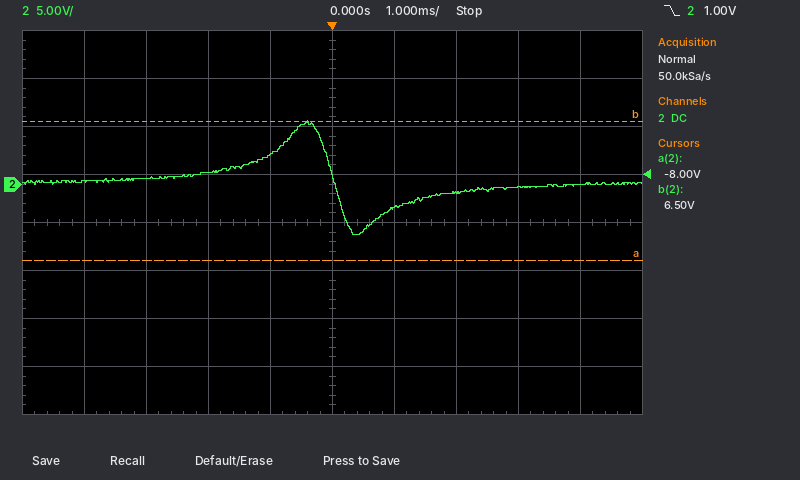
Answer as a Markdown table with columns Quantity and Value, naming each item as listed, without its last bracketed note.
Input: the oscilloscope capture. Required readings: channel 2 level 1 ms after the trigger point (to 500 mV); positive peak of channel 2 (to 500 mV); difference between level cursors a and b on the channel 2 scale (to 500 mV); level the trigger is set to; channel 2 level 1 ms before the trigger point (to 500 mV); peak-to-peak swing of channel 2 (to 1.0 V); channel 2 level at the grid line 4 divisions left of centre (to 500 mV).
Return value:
| Quantity | Value |
|---|---|
| channel 2 level 1 ms after the trigger point | -2.5 V |
| positive peak of channel 2 | 6.5 V |
| difference between level cursors a and b on the channel 2 scale | 14.5 V |
| level the trigger is set to | 1.00 V |
| channel 2 level 1 ms before the trigger point | 3.0 V |
| peak-to-peak swing of channel 2 | 12.0 V |
| channel 2 level at the grid line 4 divisions left of centre | 500 mV |
